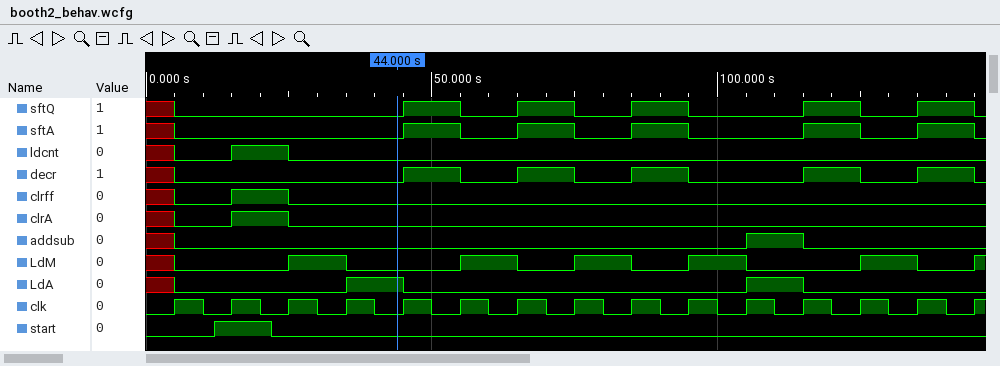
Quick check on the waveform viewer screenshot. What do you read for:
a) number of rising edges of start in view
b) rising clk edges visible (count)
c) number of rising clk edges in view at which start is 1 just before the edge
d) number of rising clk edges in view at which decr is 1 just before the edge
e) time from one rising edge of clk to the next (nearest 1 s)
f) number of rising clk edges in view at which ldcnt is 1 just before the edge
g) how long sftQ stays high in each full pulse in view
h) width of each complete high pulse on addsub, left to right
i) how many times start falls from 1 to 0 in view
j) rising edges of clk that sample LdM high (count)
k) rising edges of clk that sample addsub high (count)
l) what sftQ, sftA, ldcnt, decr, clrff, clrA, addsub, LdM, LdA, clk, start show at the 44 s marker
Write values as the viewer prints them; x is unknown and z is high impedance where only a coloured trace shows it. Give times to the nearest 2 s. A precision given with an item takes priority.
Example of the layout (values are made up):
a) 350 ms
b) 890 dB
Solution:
a) 1
b) 15
c) 1
d) 5
e) 10 s
f) 1
g) 10 s, 10 s, 10 s, 10 s, 10 s
h) 10 s
i) 1
j) 5
k) 1
l) sftQ=0, sftA=0, ldcnt=0, decr=0, clrff=0, clrA=0, addsub=0, LdM=0, LdA=1, clk=0, start=0
